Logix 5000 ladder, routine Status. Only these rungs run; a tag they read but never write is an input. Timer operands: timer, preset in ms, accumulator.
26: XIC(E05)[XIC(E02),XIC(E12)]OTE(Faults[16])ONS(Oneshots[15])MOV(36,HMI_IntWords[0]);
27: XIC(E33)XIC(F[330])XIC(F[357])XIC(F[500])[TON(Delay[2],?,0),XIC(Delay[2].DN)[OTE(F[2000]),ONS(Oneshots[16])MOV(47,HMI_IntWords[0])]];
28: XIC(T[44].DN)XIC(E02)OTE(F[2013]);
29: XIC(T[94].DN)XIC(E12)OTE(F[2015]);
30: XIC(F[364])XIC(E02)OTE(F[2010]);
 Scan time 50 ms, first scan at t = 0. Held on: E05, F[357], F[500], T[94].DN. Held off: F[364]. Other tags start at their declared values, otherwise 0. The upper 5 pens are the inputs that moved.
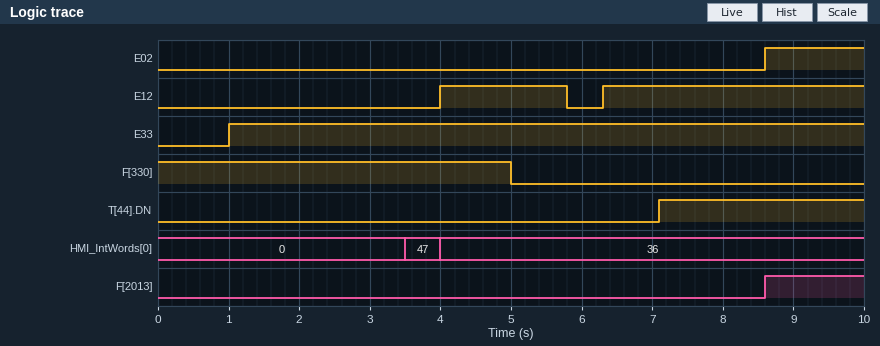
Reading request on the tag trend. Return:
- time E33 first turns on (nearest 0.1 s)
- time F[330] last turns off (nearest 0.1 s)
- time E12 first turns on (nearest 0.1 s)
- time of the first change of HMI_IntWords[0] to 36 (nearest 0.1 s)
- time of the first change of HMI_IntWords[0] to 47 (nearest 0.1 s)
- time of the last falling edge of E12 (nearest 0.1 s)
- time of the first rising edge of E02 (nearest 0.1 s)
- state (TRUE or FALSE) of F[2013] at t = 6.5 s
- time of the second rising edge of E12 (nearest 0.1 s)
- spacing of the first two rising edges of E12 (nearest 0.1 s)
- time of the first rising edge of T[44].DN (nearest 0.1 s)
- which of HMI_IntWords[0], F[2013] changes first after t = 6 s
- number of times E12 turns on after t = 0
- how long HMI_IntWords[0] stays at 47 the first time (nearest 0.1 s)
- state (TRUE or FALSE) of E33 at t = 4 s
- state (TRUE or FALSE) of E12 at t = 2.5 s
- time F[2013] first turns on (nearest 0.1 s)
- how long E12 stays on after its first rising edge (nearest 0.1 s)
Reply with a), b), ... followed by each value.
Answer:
a) 1.0 s
b) 5.0 s
c) 4.0 s
d) 4.0 s
e) 3.5 s
f) 5.8 s
g) 8.6 s
h) FALSE
i) 6.3 s
j) 2.3 s
k) 7.1 s
l) F[2013]
m) 2
n) 0.5 s
o) TRUE
p) FALSE
q) 8.6 s
r) 1.8 s
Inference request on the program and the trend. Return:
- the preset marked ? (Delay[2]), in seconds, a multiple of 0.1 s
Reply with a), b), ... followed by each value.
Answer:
a) 2.5 s
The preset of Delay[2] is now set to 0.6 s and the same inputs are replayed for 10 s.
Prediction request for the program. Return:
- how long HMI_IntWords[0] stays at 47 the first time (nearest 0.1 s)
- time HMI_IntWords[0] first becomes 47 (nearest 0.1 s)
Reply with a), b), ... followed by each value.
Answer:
a) 2.4 s
b) 1.6 s
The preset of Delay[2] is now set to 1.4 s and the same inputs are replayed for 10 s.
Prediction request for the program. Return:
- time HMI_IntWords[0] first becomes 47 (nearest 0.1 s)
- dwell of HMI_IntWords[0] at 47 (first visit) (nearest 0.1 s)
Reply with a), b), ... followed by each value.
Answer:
a) 2.4 s
b) 1.6 s
